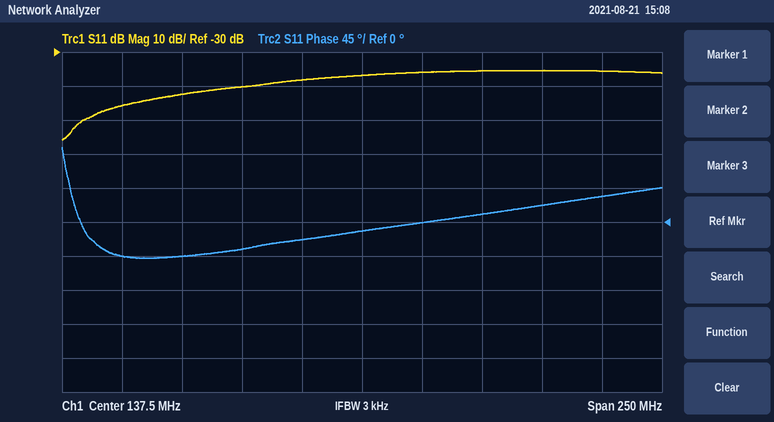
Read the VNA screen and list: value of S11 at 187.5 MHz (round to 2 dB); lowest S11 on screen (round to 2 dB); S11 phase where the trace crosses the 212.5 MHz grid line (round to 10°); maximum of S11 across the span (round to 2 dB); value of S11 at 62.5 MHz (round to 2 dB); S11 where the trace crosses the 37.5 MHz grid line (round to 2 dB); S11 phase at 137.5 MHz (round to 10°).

-36 dB
-56 dB
20°
-36 dB
-42 dB
-46 dB
-10°
